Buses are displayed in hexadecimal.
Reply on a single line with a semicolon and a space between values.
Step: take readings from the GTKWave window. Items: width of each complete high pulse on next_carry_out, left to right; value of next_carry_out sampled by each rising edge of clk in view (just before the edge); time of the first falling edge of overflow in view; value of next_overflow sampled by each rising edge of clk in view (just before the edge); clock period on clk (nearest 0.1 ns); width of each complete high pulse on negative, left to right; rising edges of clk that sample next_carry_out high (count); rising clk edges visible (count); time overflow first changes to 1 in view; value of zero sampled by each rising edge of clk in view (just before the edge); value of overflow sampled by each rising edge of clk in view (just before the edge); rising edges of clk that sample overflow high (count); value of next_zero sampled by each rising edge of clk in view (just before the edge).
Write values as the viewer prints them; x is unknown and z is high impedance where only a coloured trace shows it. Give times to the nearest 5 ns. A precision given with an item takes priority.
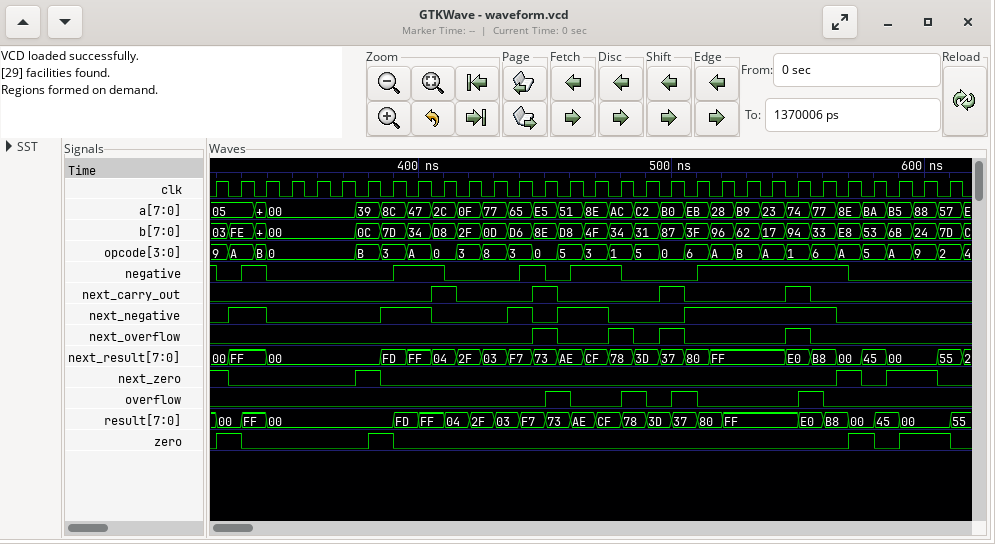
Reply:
10 ns, 10 ns, 10 ns, 10 ns; 0 0 0 0 0 0 0 0 0 1 0 0 0 1 0 0 0 0 1 0 0 0 0 1 0 0 0 0 0 0; 460 ns; 0 0 0 0 0 0 0 0 0 0 0 0 0 1 0 0 1 0 1 0 0 0 0 1 0 0 0 0 0 0; 10 ns; 10 ns, 20 ns, 10 ns, 20 ns, 60 ns; 4; 30; 450 ns; 0 1 0 0 0 0 0 1 0 0 0 0 0 0 0 0 0 0 0 0 0 0 0 0 0 0 1 0 1 1; 0 0 0 0 0 0 0 0 0 0 0 0 0 0 1 0 0 1 0 1 0 0 0 0 1 0 0 0 0 0; 4; 1 0 0 0 0 0 1 0 0 0 0 0 0 0 0 0 0 0 0 0 0 0 0 0 0 1 0 1 1 0
